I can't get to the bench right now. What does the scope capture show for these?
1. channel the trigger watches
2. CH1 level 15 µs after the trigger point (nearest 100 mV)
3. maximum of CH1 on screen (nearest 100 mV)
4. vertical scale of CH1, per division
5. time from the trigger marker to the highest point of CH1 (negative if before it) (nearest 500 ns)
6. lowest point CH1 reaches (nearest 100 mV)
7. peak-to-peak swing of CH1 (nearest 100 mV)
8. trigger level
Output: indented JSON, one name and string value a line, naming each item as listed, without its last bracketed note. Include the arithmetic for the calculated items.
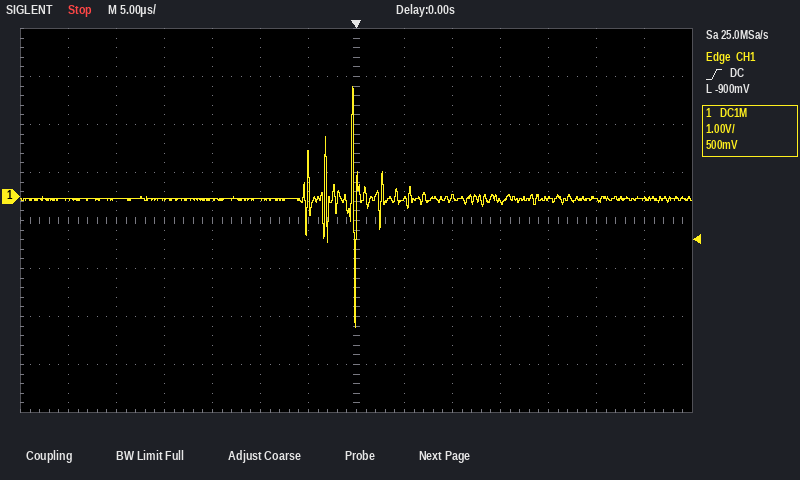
{
  "channel the trigger watches": "CH1",
  "CH1 level 15 µs after the trigger point": "-100 mV",
  "maximum of CH1 on screen": "2.3 V",
  "vertical scale of CH1, per division": "1 V",
  "time from the trigger marker to the highest point of CH1 (negative if before it)": "-500 ns",
  "lowest point CH1 reaches": "-2.7 V",
  "peak-to-peak swing of CH1": "2.3 V − (-2.7 V) = 5.0 V",
  "trigger level": "-900 mV"
}
